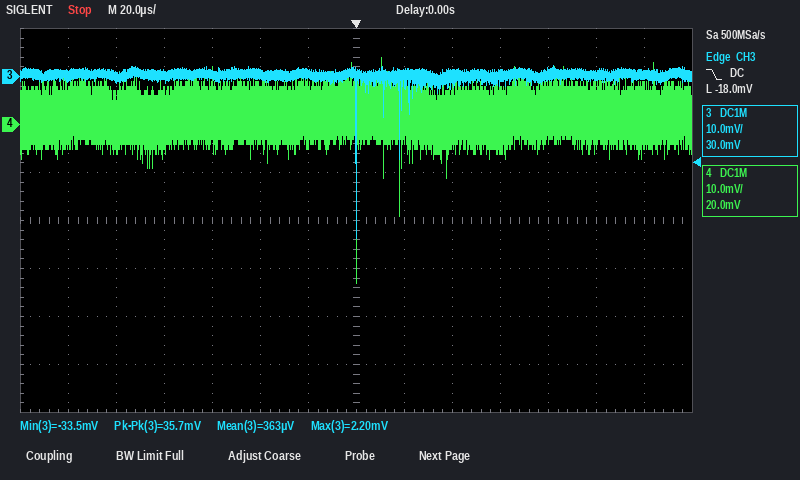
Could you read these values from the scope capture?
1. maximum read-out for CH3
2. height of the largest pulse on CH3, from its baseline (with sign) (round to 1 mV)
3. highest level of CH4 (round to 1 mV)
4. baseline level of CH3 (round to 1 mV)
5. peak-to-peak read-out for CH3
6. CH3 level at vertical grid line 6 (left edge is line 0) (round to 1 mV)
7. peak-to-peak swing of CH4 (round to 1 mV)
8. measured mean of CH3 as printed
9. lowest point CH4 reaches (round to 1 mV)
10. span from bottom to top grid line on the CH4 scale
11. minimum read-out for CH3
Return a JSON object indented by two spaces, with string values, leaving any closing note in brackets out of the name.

{
  "maximum read-out for CH3": "2.20 mV",
  "height of the largest pulse on CH3, from its baseline (with sign)": "-34 mV",
  "highest level of CH4": "14 mV",
  "baseline level of CH3": "0 mV",
  "peak-to-peak read-out for CH3": "35.7 mV",
  "CH3 level at vertical grid line 6 (left edge is line 0)": "1 mV",
  "peak-to-peak swing of CH4": "47 mV",
  "measured mean of CH3 as printed": "363 µV",
  "lowest point CH4 reaches": "-33 mV",
  "span from bottom to top grid line on the CH4 scale": "80 mV",
  "minimum read-out for CH3": "-33.5 mV"
}
